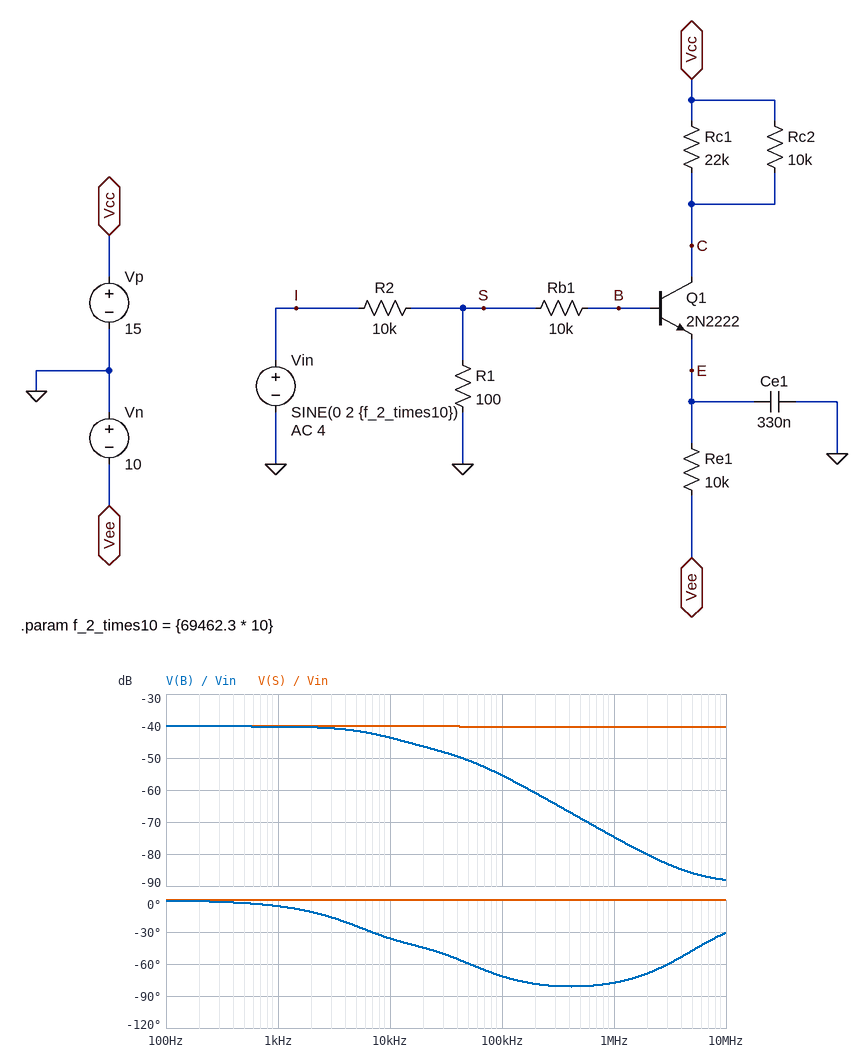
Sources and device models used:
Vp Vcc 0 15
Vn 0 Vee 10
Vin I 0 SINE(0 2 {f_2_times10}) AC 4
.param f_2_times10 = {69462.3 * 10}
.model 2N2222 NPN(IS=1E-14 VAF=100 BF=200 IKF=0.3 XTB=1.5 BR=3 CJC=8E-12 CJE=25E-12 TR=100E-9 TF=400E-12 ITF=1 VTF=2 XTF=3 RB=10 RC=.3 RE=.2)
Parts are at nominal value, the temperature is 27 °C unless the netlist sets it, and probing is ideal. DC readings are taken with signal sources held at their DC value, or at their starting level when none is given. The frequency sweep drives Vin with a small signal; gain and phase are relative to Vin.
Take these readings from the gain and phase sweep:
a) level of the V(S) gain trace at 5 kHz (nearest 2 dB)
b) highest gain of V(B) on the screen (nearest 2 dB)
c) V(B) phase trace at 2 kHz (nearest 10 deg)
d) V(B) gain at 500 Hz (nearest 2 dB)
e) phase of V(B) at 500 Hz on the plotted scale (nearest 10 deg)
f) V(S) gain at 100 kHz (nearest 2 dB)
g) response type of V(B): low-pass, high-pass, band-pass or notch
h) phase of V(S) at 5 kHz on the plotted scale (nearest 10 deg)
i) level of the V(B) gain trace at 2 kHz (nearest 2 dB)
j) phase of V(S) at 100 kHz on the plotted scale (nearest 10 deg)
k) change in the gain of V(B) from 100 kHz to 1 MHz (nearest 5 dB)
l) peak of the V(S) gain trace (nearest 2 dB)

-40 dB
-40 dB
-10 deg
-40 dB
0 deg
-40 dB
low-pass
0 deg
-40 dB
0 deg
-20 dB
-40 dB
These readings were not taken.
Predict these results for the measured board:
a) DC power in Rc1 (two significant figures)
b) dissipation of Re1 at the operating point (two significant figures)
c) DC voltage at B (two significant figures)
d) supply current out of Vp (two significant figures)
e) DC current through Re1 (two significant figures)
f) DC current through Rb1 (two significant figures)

1.8 mW
8.7 mW
-43 mV
930 µA
930 µA
4.3 µA
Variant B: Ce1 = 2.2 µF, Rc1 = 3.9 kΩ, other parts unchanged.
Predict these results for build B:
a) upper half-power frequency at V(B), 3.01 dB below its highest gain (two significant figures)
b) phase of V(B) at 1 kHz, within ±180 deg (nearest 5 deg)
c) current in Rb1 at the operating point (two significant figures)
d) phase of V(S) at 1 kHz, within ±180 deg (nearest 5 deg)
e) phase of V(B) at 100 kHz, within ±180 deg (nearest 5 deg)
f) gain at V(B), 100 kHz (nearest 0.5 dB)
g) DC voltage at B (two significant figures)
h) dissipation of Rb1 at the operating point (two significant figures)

1.2 kHz
-25 deg
4.1 µA
0 deg
-40 deg
-51.0 dB
-42 mV
170 nW
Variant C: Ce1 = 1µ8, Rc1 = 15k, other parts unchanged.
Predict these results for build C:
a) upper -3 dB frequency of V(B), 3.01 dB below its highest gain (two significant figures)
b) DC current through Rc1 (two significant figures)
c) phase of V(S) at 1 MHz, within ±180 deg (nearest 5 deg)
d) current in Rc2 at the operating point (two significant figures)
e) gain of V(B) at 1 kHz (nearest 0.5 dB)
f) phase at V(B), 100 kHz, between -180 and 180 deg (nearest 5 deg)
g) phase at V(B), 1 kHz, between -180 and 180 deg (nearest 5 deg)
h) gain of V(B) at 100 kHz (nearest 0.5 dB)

1.4 kHz
370 µA
0 deg
560 µA
-42.0 dB
-60 deg
-25 deg
-54.5 dB
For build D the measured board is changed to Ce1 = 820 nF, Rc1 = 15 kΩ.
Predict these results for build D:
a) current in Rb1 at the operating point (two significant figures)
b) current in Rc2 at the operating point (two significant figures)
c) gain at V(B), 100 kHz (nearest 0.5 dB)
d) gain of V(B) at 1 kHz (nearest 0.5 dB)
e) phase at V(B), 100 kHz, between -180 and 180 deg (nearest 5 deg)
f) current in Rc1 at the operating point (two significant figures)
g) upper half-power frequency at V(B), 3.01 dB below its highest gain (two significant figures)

4.2 µA
560 µA
-54.5 dB
-40.5 dB
-65 deg
370 µA
3.2 kHz
